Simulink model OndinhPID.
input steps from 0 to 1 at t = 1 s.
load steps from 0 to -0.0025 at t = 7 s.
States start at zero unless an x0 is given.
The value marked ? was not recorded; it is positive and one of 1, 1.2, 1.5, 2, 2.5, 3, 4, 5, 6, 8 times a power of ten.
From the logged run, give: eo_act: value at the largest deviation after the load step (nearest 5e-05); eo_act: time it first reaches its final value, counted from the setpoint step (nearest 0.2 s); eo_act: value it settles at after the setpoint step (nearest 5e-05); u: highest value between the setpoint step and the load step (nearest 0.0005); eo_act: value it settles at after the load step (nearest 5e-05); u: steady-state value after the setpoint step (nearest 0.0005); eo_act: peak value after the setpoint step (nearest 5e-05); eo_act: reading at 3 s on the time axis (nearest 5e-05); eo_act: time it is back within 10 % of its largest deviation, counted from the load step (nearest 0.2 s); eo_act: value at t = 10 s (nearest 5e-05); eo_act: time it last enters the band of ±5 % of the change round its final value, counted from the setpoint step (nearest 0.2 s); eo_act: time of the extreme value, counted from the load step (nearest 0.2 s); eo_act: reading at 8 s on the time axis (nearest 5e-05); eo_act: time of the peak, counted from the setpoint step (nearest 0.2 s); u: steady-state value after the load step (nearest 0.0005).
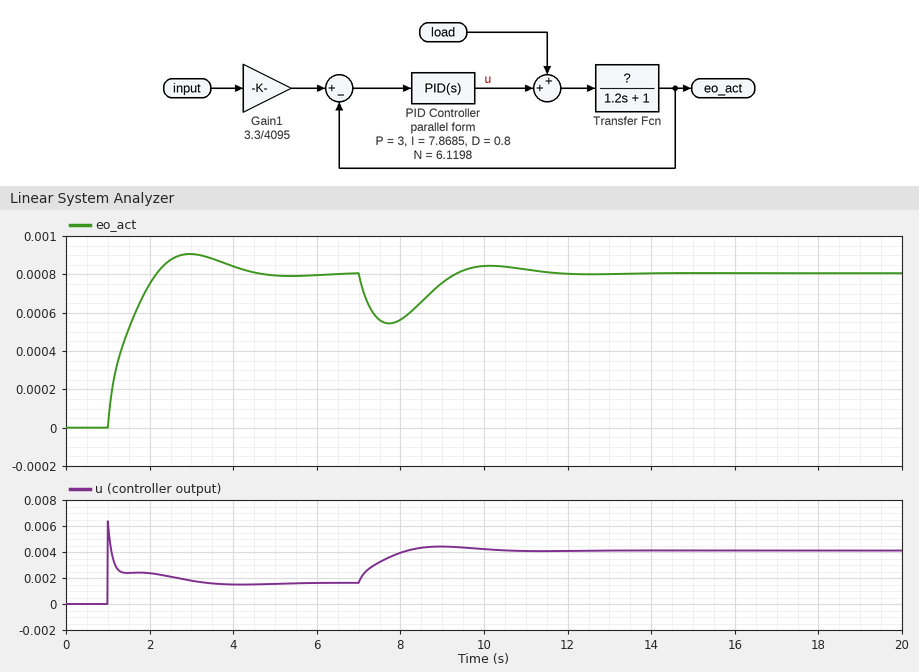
0.00055
1.2 s
0.00080
0.0065
0.00080
0.0015
0.00090
0.00090
3.8 s
0.00085
3.0 s
0.8 s
0.00055
2.0 s
0.0040
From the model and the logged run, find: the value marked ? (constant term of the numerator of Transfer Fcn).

0.5
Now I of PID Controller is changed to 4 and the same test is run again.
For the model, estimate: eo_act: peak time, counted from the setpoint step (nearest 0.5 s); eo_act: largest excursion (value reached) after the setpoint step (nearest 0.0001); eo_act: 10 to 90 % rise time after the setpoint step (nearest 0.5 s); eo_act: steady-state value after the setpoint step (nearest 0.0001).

3.0 s
0.0008
1.5 s
0.0008
